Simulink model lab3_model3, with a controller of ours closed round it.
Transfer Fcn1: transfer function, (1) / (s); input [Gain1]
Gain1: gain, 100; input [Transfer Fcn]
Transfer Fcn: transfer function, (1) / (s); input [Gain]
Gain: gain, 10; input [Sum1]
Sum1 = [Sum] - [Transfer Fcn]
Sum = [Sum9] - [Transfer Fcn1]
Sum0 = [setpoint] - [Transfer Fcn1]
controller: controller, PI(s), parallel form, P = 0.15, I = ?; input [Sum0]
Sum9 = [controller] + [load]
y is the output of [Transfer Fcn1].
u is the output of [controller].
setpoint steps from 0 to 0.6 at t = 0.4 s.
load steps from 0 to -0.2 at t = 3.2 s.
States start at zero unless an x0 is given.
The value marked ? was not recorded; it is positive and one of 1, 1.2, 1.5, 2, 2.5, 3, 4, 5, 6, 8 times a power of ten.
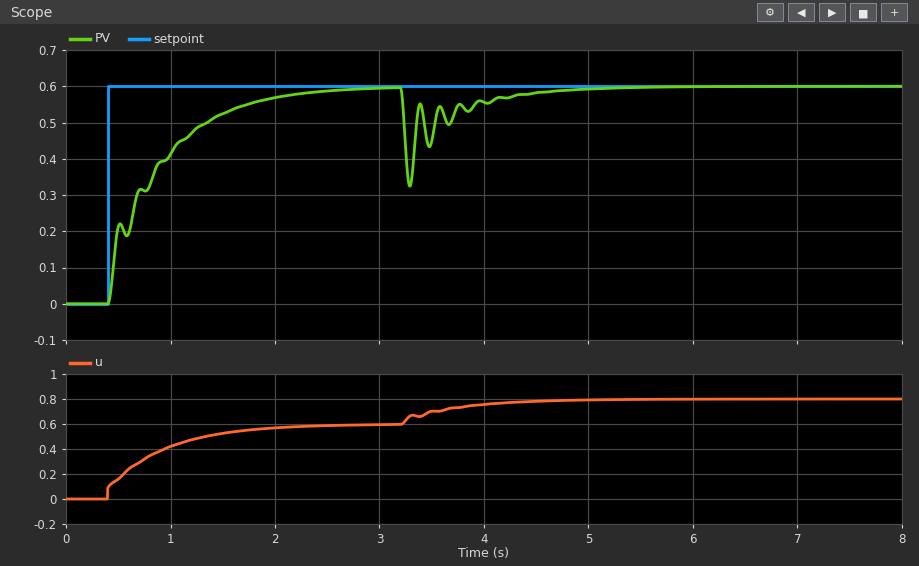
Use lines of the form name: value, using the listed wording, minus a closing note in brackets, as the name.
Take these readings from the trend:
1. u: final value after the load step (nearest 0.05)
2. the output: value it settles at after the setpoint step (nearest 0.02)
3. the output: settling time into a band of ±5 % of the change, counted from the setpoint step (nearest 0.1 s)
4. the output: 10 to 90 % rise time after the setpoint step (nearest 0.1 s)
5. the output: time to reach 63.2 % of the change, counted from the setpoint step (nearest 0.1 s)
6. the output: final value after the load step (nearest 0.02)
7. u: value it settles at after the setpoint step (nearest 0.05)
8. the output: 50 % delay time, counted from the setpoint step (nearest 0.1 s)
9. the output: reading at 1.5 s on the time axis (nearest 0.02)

u: final value after the load step: 0.80
the output: value it settles at after the setpoint step: 0.60
the output: settling time into a band of ±5 % of the change, counted from the setpoint step: 1.6 s
the output: 10 to 90 % rise time after the setpoint step: 1.2 s
the output: time to reach 63.2 % of the change, counted from the setpoint step: 0.5 s
the output: final value after the load step: 0.60
u: value it settles at after the setpoint step: 0.60
the output: 50 % delay time, counted from the setpoint step: 0.3 s
the output: reading at 1.5 s on the time axis: 0.52
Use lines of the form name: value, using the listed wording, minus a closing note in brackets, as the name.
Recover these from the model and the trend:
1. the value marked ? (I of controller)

the value marked ?: 2
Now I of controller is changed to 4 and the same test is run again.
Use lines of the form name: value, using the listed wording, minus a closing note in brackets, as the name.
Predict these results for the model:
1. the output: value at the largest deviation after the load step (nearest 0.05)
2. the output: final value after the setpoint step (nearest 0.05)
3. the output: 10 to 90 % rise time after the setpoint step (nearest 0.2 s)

the output: value at the largest deviation after the load step: 0.35
the output: final value after the setpoint step: 0.60
the output: 10 to 90 % rise time after the setpoint step: 0.6 s
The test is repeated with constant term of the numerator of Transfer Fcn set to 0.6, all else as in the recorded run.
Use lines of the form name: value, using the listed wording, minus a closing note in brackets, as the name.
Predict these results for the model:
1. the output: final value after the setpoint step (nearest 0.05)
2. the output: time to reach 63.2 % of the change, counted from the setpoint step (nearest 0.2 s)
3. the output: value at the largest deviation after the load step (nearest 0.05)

the output: final value after the setpoint step: 0.60
the output: time to reach 63.2 % of the change, counted from the setpoint step: 0.6 s
the output: value at the largest deviation after the load step: 0.30
